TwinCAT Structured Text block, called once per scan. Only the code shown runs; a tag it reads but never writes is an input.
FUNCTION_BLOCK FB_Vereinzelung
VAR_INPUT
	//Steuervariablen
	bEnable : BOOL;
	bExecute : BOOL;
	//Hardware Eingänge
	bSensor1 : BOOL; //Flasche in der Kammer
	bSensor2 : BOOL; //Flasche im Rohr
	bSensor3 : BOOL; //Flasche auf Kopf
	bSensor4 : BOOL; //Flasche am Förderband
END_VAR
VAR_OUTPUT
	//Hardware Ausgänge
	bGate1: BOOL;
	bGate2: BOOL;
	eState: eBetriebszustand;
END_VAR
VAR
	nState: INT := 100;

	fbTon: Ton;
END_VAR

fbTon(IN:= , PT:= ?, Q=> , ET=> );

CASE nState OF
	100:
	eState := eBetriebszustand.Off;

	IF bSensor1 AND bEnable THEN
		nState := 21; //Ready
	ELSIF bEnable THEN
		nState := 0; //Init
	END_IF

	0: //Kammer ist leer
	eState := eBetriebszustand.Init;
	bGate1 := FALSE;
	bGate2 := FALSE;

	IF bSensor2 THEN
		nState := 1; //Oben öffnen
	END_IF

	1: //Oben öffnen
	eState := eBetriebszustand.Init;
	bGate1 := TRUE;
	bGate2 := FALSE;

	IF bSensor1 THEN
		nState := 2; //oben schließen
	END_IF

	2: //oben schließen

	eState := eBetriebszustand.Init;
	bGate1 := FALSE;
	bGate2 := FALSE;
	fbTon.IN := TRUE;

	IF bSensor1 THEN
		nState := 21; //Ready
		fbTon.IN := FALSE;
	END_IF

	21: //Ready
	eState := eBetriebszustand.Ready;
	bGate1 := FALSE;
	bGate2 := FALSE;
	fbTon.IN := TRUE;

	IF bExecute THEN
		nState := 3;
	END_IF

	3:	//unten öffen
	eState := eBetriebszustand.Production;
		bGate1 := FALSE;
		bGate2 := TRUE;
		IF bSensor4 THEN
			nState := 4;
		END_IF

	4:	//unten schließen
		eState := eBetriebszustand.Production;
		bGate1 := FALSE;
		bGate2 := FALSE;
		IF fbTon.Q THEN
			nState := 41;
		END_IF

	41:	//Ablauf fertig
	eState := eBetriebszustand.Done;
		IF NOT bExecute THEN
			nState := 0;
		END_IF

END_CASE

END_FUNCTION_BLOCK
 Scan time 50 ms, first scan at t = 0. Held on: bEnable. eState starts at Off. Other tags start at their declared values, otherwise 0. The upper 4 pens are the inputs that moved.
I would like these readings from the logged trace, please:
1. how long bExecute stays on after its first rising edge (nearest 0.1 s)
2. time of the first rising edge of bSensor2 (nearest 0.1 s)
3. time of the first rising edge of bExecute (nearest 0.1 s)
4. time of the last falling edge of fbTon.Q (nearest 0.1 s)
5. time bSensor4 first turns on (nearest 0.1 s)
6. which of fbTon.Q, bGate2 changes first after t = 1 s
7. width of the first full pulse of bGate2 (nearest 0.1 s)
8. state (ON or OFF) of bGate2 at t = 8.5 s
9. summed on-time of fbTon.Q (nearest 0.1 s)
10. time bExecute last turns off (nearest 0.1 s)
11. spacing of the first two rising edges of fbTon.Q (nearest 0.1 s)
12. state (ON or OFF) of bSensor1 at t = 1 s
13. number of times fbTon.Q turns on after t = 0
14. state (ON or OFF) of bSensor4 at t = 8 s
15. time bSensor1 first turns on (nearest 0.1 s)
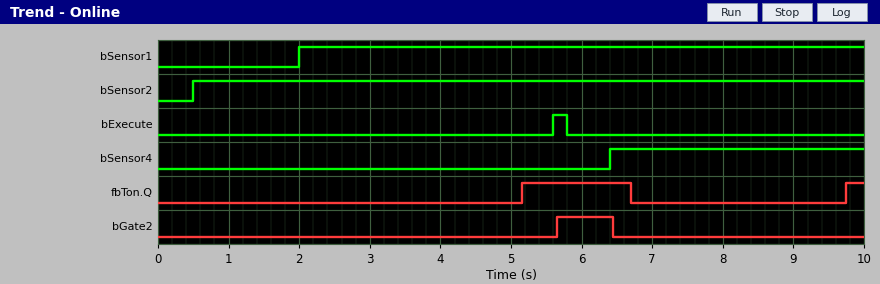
0.2 s
0.5 s
5.6 s
6.7 s
6.4 s
fbTon.Q
0.8 s
OFF
1.8 s
5.8 s
4.6 s
OFF
2
ON
2.0 s
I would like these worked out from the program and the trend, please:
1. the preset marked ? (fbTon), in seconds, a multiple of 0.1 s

3.0 s
